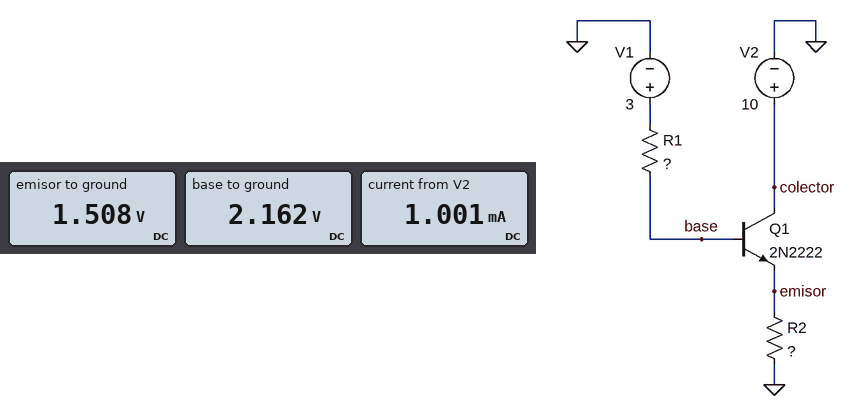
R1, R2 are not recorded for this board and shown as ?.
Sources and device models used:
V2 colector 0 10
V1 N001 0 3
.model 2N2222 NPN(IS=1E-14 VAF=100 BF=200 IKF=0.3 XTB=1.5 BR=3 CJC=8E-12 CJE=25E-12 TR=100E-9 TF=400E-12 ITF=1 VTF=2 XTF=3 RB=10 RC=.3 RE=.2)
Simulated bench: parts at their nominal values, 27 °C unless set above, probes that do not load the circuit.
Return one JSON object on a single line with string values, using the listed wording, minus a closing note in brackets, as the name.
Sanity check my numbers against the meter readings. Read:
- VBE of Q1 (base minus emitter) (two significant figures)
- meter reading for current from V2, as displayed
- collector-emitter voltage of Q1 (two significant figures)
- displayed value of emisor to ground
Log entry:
{"VBE of Q1 (base minus emitter)": "650 mV", "meter reading for current from V2, as displayed": "1.001 mA", "collector-emitter voltage of Q1": "8.5 V", "displayed value of emisor to ground": "1.508 V"}
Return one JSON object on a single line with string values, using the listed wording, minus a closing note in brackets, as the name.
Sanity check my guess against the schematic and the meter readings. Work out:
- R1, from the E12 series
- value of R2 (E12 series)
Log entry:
{"R1, from the E12 series": "180 kΩ", "value of R2": "1.5 kΩ"}
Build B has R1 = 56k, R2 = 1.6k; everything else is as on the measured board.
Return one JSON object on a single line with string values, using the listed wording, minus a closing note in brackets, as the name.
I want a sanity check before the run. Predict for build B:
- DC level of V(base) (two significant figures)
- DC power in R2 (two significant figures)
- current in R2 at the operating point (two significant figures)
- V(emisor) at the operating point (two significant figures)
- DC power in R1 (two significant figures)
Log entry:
{"DC level of V(base)": "2.7 V", "DC power in R2": "2.5 mW", "current in R2 at the operating point": "1.3 mA", "V(emisor) at the operating point": "2.0 V", "DC power in R1": "1.9 µW"}
